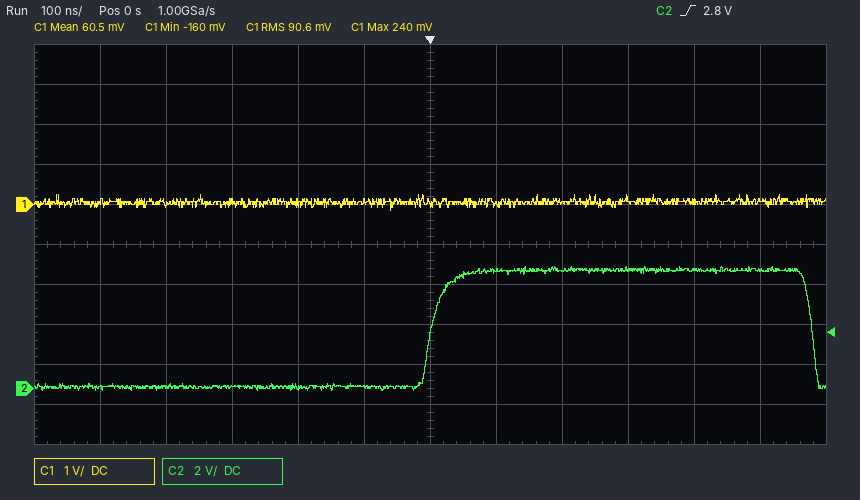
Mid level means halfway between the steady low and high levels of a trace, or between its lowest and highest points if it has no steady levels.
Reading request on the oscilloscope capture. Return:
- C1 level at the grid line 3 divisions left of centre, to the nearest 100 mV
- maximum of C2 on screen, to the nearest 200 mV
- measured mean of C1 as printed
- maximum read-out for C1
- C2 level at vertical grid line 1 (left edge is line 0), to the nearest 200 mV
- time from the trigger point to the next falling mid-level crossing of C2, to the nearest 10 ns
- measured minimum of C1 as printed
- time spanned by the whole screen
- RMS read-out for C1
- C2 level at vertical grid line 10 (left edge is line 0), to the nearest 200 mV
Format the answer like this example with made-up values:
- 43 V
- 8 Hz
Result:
- 100 mV
- 6.0 V
- 60.5 mV
- 240 mV
- 0.0 V
- 580 ns
- -160 mV
- 1.2 µs
- 90.6 mV
- 6.0 V
